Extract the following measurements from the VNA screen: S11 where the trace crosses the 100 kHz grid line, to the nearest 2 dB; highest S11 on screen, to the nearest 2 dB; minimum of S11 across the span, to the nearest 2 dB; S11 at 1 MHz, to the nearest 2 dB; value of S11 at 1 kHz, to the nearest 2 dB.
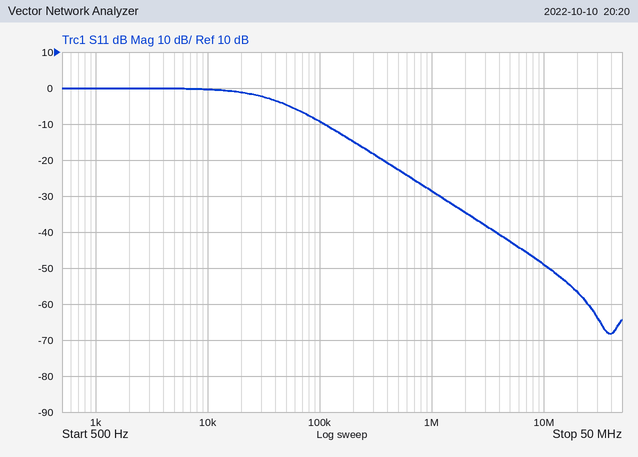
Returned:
-10 dB
0 dB
-68 dB
-28 dB
0 dB
